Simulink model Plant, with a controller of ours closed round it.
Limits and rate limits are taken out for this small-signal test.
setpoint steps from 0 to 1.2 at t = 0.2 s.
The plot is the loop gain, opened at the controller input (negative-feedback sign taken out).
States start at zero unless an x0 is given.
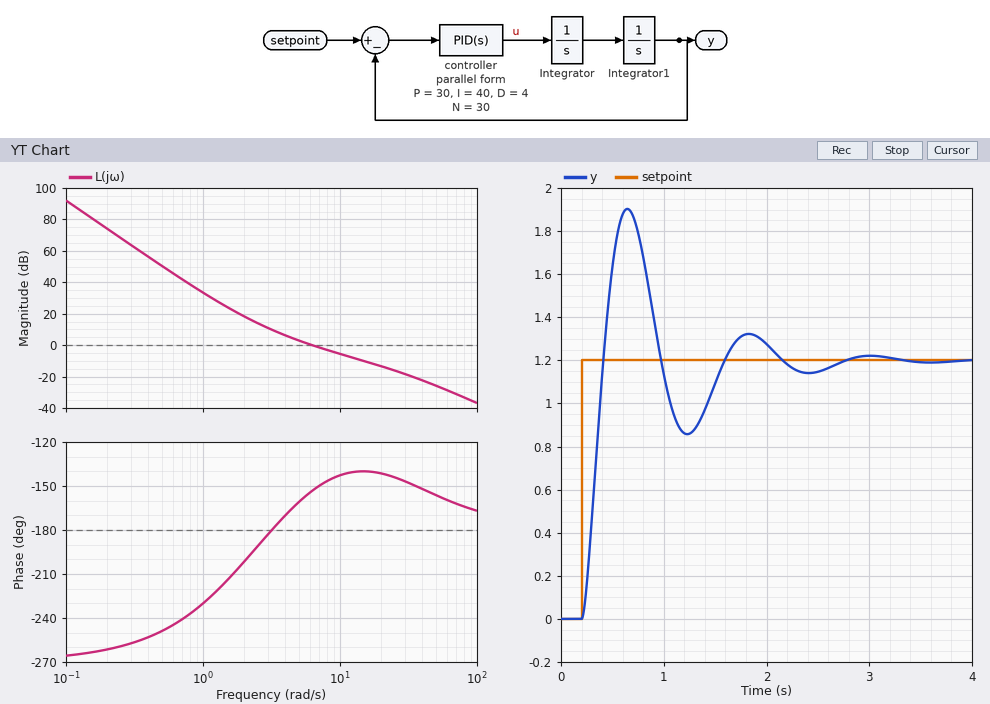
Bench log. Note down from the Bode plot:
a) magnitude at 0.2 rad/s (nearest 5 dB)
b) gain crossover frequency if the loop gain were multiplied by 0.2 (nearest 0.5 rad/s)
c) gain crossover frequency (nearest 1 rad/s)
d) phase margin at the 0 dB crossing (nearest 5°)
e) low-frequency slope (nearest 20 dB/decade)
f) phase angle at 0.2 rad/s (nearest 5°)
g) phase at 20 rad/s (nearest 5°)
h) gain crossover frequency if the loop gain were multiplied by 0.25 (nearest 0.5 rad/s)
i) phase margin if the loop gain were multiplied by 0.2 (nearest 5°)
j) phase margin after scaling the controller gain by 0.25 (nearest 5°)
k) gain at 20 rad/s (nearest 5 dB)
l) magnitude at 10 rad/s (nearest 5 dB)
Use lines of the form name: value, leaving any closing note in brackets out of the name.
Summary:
magnitude at 0.2 rad/s: 75 dB
gain crossover frequency if the loop gain were multiplied by 0.2: 2.5 rad/s
gain crossover frequency: 6 rad/s
phase margin at the 0 dB crossing: 25°
low-frequency slope: -60 dB/decade
phase angle at 0.2 rad/s: -260°
phase at 20 rad/s: -140°
gain crossover frequency if the loop gain were multiplied by 0.25: 3.0 rad/s
phase margin if the loop gain were multiplied by 0.2: -10°
phase margin after scaling the controller gain by 0.25: -5°
gain at 20 rad/s: -15 dB
magnitude at 10 rad/s: -5 dB
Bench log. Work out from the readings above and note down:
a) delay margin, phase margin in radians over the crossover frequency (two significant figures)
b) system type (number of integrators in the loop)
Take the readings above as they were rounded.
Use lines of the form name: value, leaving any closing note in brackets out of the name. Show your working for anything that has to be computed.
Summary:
delay margin, phase margin in radians over the crossover frequency: 25 × π / 180 / 6 = 0.073 s
system type: 3
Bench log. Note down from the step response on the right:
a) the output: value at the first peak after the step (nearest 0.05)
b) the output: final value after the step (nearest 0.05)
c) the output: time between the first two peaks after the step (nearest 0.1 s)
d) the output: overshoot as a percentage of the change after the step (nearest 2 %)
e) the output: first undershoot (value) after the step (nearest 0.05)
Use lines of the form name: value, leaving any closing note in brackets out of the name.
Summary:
the output: value at the first peak after the step: 1.90
the output: final value after the step: 1.20
the output: time between the first two peaks after the step: 1.2 s
the output: overshoot as a percentage of the change after the step: 58 %
the output: first undershoot (value) after the step: 0.85
